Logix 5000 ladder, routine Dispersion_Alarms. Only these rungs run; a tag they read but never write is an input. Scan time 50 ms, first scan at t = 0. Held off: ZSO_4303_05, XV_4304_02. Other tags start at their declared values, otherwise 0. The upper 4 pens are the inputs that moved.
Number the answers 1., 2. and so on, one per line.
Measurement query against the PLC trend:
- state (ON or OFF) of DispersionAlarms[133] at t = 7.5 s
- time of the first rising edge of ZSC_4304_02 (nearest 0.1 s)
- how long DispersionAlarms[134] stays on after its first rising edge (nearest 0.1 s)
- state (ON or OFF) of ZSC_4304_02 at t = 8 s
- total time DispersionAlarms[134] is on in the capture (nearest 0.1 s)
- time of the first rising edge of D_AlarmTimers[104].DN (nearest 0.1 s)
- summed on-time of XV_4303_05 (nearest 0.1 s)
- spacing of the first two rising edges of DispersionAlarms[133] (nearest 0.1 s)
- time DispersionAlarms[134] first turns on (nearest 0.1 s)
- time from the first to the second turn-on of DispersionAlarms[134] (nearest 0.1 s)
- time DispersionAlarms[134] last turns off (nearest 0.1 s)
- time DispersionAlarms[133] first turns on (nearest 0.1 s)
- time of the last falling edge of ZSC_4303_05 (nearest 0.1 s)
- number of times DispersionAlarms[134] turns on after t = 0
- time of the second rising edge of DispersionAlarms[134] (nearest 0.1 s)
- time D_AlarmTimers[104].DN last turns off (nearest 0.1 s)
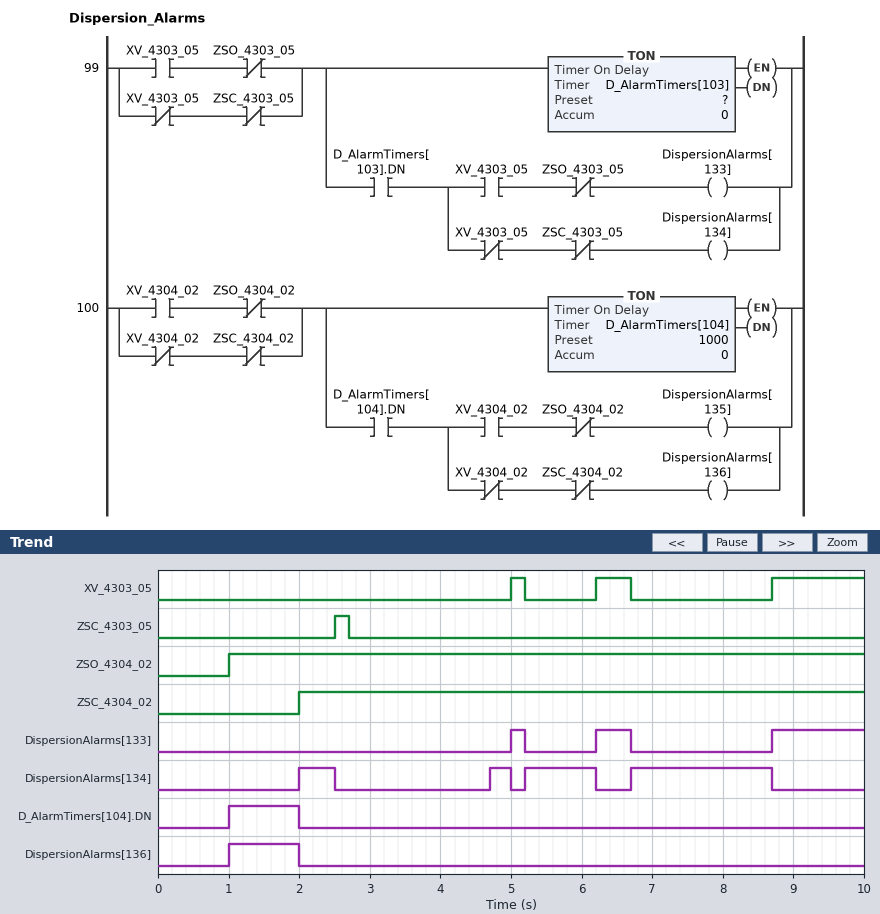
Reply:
1. OFF
2. 2.0 s
3. 0.5 s
4. ON
5. 3.8 s
6. 1.0 s
7. 2.0 s
8. 1.2 s
9. 2.0 s
10. 2.7 s
11. 8.7 s
12. 5.0 s
13. 2.7 s
14. 4
15. 4.7 s
16. 2.0 s
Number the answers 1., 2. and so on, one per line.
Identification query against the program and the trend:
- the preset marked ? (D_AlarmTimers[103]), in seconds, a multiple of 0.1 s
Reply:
1. 2.0 s
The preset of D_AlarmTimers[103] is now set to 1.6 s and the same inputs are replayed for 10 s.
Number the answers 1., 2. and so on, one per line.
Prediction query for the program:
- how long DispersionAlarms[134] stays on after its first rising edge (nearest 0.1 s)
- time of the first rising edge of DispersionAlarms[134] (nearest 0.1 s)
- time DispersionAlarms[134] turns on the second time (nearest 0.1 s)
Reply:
1. 0.9 s
2. 1.6 s
3. 4.3 s
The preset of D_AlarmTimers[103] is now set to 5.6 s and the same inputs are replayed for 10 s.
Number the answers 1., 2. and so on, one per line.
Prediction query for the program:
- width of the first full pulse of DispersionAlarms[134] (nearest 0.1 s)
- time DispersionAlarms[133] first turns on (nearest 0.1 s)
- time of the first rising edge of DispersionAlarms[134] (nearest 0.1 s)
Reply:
1. 0.4 s
2. 8.7 s
3. 8.3 s
